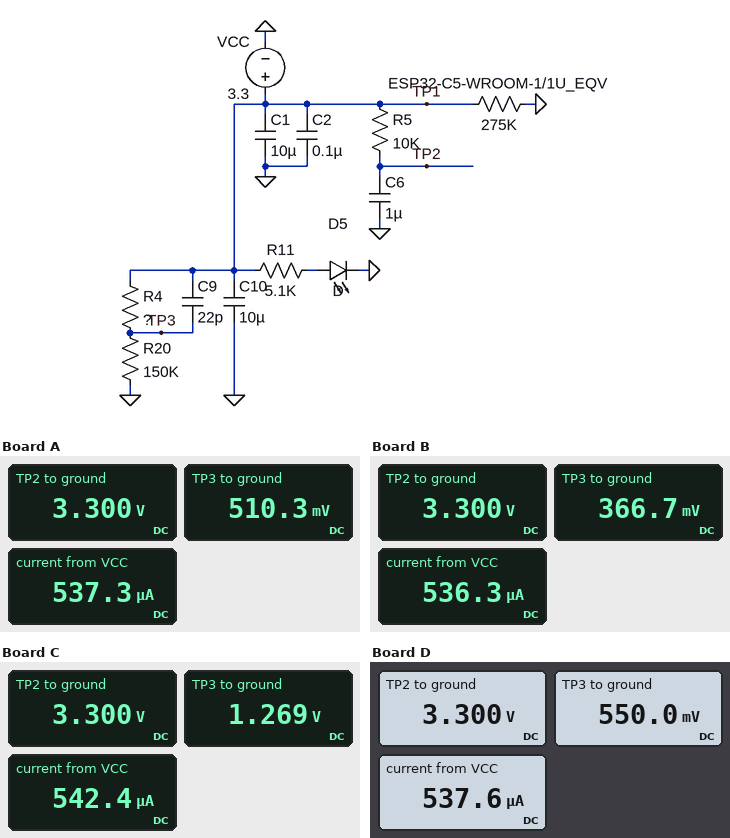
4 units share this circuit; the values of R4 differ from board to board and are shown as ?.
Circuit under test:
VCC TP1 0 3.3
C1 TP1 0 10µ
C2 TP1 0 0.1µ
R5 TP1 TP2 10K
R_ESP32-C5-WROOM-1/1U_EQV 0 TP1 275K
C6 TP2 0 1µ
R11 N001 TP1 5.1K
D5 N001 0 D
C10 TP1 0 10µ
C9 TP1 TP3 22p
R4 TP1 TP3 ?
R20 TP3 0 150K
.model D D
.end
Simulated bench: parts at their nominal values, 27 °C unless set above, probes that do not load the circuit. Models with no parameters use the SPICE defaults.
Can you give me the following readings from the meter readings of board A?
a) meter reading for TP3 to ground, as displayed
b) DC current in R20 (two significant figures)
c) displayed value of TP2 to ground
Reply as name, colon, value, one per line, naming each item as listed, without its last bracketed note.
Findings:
meter reading for TP3 to ground, as displayed: 510.3 mV
DC current in R20: 3.4 µA
displayed value of TP2 to ground: 3.300 V
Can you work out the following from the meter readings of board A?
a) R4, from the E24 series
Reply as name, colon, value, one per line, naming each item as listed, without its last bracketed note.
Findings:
R4, from the E24 series: 820 kΩ
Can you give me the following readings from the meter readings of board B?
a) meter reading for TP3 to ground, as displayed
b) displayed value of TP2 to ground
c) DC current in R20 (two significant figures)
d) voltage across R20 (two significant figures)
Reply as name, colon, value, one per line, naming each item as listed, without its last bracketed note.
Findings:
meter reading for TP3 to ground, as displayed: 366.7 mV
displayed value of TP2 to ground: 3.300 V
DC current in R20: 2.4 µA
voltage across R20: 370 mV
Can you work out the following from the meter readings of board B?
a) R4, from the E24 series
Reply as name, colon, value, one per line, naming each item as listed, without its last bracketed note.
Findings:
R4, from the E24 series: 1.2 MΩ
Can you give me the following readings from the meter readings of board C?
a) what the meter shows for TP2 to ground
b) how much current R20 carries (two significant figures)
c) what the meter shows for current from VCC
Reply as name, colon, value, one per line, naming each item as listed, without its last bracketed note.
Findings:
what the meter shows for TP2 to ground: 3.300 V
how much current R20 carries: 8.5 µA
what the meter shows for current from VCC: 542.4 µA
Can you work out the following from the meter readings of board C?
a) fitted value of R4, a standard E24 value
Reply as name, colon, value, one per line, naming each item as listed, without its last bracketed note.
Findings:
fitted value of R4, a standard E24 value: 240 kΩ
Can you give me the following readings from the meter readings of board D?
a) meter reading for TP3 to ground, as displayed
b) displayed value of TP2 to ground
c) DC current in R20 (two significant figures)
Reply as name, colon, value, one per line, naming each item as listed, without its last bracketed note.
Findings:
meter reading for TP3 to ground, as displayed: 550.0 mV
displayed value of TP2 to ground: 3.300 V
DC current in R20: 3.7 µA
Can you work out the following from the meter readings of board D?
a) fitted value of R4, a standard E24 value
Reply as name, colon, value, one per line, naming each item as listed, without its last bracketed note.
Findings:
fitted value of R4, a standard E24 value: 750 kΩ
